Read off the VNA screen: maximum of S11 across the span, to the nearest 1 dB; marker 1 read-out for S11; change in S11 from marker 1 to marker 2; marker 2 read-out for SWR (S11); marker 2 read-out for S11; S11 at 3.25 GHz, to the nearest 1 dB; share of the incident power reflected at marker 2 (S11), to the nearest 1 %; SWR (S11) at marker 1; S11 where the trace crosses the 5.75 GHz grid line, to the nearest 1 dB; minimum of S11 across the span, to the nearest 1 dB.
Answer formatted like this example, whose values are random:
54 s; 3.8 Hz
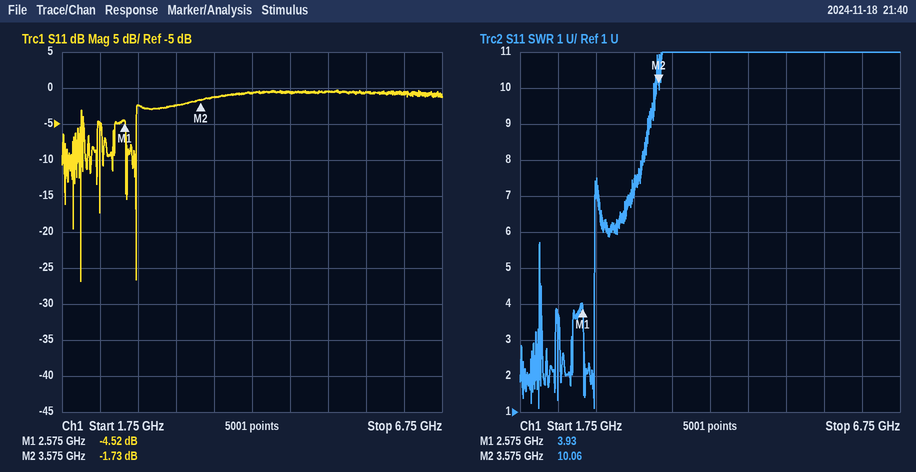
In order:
0 dB; -4.52 dB; 2.79 dB; 10.06; -1.73 dB; -2 dB; 67 %; 3.93; -1 dB; -27 dB
